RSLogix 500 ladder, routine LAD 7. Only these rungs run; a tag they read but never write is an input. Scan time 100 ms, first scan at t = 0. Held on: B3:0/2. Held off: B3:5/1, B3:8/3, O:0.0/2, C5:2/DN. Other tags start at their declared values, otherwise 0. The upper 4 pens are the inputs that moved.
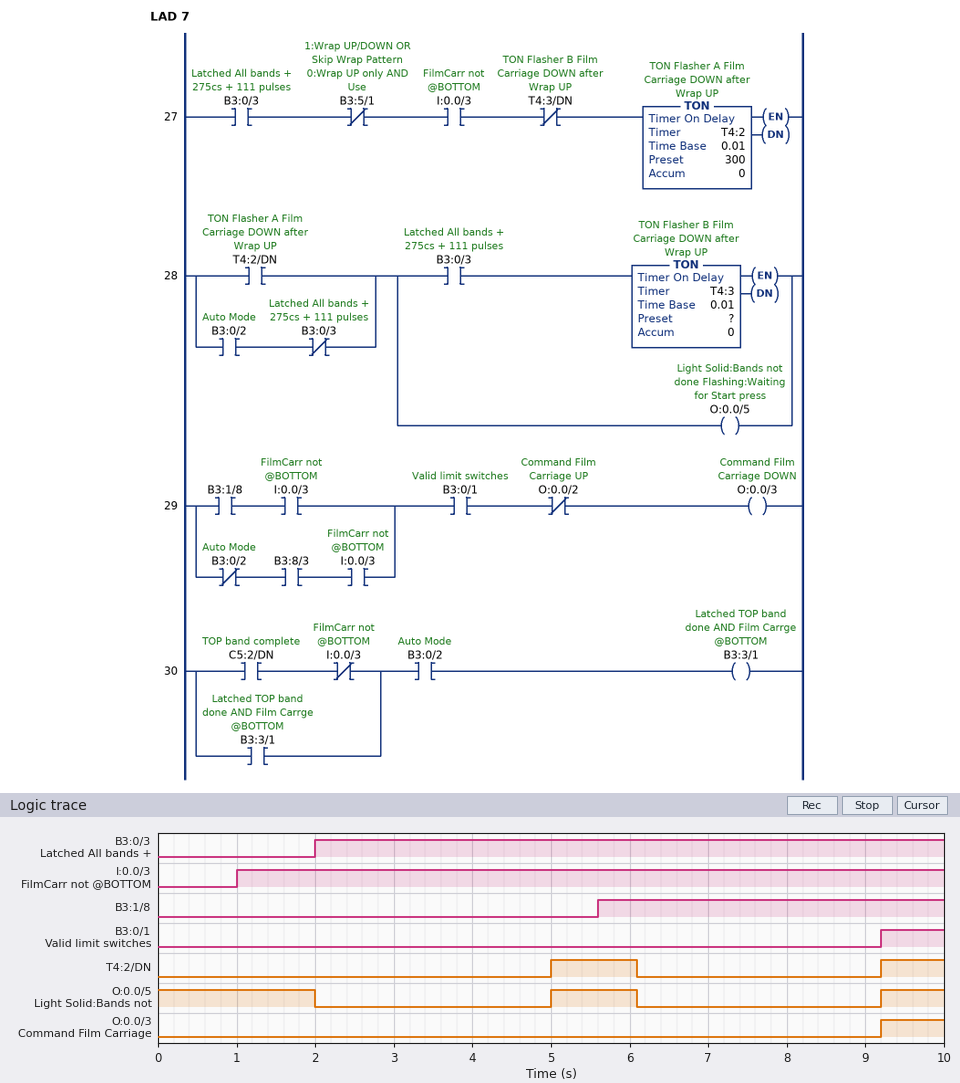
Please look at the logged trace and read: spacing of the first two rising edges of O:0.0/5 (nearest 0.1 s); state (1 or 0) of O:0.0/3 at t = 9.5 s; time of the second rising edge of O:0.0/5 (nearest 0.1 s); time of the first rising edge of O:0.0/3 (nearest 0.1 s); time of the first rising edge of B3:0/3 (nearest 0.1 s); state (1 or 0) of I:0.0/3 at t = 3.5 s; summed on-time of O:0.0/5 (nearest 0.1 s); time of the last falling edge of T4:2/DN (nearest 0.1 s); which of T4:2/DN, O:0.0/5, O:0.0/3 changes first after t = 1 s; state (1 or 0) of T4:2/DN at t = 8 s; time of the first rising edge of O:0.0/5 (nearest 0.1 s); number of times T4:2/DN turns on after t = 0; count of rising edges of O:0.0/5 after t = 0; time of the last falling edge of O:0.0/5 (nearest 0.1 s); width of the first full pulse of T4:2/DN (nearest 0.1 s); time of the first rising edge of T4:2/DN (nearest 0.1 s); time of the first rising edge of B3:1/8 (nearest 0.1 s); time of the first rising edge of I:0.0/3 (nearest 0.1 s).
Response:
4.2 s
1
9.2 s
9.2 s
2.0 s
1
3.9 s
6.1 s
O:0.0/5
0
5.0 s
2
2
6.1 s
1.1 s
5.0 s
5.6 s
1.0 s
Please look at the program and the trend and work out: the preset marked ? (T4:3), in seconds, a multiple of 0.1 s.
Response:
1.0 s
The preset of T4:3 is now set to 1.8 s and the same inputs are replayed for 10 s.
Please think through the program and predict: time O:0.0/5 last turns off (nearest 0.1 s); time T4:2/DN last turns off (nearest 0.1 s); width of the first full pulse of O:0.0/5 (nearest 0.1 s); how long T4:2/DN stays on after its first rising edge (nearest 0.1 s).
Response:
6.9 s
6.9 s
1.9 s
1.9 s
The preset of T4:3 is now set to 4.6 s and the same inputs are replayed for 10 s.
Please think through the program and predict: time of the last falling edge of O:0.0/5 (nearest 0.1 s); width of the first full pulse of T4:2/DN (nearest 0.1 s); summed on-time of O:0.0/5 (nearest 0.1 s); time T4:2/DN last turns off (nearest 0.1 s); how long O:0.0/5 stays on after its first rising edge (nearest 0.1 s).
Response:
9.7 s
4.7 s
6.7 s
9.7 s
4.7 s
